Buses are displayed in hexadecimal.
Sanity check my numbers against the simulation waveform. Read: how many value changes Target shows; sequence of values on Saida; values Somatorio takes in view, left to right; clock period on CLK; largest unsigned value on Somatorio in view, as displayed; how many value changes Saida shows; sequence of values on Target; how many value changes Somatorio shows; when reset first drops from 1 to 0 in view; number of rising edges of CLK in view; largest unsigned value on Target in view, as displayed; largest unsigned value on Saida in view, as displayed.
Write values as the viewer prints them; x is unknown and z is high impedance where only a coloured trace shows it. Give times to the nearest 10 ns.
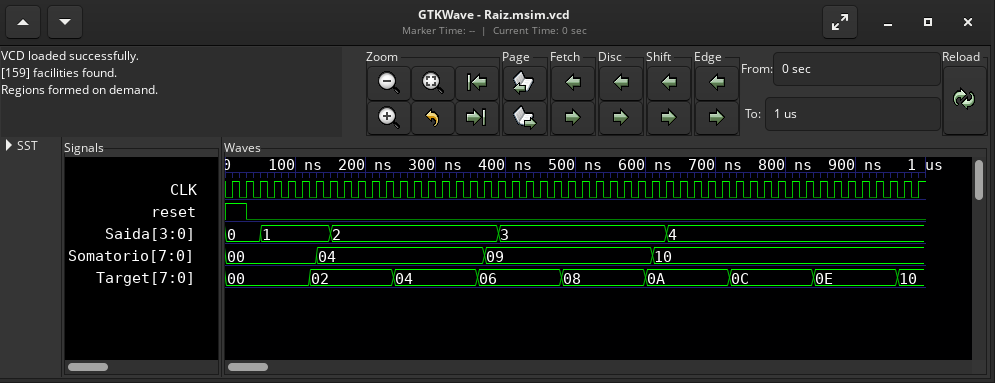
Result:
8
0, 1, 2, 3, 4
00, 04, 09, 10
20 ns
10
4
00, 02, 04, 06, 08, 0A, 0C, 0E, 10
3
30 ns
50
10
4
